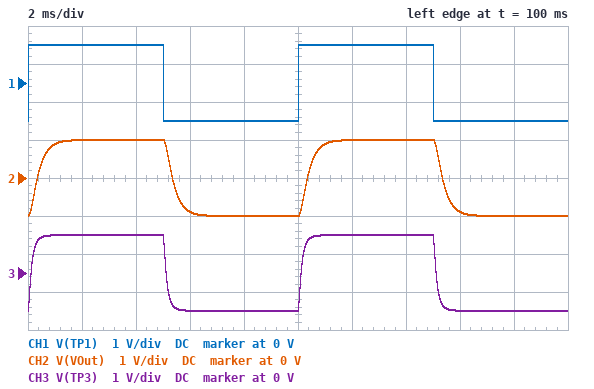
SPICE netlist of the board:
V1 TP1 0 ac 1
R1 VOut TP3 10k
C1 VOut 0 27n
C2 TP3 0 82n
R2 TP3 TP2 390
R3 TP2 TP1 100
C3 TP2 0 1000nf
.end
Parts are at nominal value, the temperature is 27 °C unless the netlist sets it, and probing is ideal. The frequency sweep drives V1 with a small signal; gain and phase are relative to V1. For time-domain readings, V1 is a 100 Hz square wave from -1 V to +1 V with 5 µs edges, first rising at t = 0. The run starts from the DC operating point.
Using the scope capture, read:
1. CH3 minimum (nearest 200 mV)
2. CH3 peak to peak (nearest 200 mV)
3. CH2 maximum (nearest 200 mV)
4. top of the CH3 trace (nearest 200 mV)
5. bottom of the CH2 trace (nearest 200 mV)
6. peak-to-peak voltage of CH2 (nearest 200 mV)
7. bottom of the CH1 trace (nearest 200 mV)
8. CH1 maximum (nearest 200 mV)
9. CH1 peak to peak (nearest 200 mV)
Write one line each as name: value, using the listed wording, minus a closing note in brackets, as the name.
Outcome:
CH3 minimum: -1.0 V
CH3 peak to peak: 2.0 V
CH2 maximum: 1.0 V
top of the CH3 trace: 1.0 V
bottom of the CH2 trace: -1.0 V
peak-to-peak voltage of CH2: 2.0 V
bottom of the CH1 trace: -1.0 V
CH1 maximum: 1.0 V
CH1 peak to peak: 2.0 V
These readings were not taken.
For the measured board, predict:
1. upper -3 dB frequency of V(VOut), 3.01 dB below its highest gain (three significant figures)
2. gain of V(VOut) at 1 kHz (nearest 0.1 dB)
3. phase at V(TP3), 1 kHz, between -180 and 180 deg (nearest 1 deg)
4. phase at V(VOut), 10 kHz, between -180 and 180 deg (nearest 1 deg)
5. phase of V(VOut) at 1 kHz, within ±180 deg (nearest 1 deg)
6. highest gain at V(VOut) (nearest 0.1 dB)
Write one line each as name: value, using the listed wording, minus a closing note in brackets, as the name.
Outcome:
upper -3 dB frequency of V(VOut), 3.01 dB below its highest gain: 491 Hz
gain of V(VOut) at 1 kHz: -8.1 dB
phase at V(TP3), 1 kHz, between -180 and 180 deg: -46 deg
phase at V(VOut), 10 kHz, between -180 and 180 deg: 131 deg
phase of V(VOut) at 1 kHz, within ±180 deg: -105 deg
highest gain at V(VOut): 0 dB
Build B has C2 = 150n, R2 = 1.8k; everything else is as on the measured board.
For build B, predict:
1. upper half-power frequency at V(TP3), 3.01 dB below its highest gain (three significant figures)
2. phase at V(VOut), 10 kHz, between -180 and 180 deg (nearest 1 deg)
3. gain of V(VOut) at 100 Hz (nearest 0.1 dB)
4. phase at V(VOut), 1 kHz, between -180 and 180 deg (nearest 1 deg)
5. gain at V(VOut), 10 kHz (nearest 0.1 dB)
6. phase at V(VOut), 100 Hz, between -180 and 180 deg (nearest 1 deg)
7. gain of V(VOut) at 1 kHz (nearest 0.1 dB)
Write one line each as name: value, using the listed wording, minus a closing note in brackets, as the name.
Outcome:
upper half-power frequency at V(TP3), 3.01 dB below its highest gain: 423 Hz
phase at V(VOut), 10 kHz, between -180 and 180 deg: 107 deg
gain of V(VOut) at 100 Hz: -0.4 dB
phase at V(VOut), 1 kHz, between -180 and 180 deg: -149 deg
gain at V(VOut), 10 kHz: -65.3 dB
phase at V(VOut), 100 Hz, between -180 and 180 deg: -25 deg
gain of V(VOut) at 1 kHz: -14.1 dB
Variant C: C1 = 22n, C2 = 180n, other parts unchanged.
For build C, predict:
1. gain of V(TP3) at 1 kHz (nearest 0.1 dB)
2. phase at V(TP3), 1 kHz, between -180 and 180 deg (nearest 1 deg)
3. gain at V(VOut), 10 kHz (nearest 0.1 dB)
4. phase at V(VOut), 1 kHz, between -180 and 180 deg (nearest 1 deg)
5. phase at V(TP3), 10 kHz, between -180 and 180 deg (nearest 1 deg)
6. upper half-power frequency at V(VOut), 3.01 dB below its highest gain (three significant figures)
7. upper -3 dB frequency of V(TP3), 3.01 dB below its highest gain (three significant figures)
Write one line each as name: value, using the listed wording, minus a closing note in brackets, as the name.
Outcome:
gain of V(TP3) at 1 kHz: -3.1 dB
phase at V(TP3), 1 kHz, between -180 and 180 deg: -59 deg
gain at V(VOut), 10 kHz: -52.2 dB
phase at V(VOut), 1 kHz, between -180 and 180 deg: -113 deg
phase at V(TP3), 10 kHz, between -180 and 180 deg: -156 deg
upper half-power frequency at V(VOut), 3.01 dB below its highest gain: 531 Hz
upper -3 dB frequency of V(TP3), 3.01 dB below its highest gain: 978 Hz
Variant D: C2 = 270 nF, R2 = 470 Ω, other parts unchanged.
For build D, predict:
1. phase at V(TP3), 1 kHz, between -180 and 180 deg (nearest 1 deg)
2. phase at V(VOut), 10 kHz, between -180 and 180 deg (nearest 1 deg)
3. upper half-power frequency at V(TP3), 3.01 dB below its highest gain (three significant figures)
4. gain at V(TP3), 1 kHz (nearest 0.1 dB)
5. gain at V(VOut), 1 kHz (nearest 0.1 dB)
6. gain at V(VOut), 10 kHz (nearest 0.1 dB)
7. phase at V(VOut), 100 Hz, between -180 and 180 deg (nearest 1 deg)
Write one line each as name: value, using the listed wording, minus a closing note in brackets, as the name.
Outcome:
phase at V(TP3), 1 kHz, between -180 and 180 deg: -72 deg
phase at V(VOut), 10 kHz, between -180 and 180 deg: 112 deg
upper half-power frequency at V(TP3), 3.01 dB below its highest gain: 721 Hz
gain at V(TP3), 1 kHz: -4.7 dB
gain at V(VOut), 1 kHz: -10.6 dB
gain at V(VOut), 10 kHz: -58.9 dB
phase at V(VOut), 100 Hz, between -180 and 180 deg: -19 deg
